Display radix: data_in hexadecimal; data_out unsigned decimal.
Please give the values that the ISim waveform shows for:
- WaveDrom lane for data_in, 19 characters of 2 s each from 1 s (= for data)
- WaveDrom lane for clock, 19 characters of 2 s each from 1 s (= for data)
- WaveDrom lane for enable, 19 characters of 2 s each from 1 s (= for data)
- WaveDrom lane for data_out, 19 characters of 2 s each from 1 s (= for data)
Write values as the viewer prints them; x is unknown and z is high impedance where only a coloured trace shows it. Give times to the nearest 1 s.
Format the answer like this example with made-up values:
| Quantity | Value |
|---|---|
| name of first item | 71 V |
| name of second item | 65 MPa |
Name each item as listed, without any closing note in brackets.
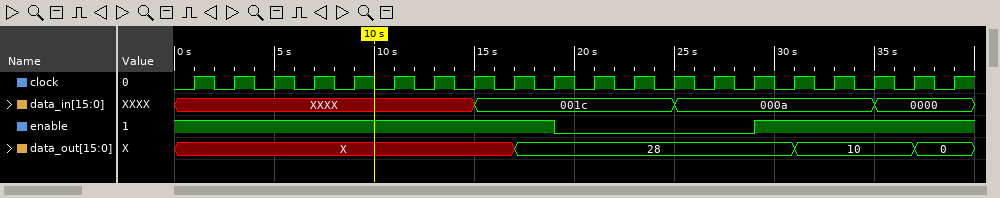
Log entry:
| Quantity | Value |
|---|---|
| WaveDrom lane for data_in, 19 characters of 2 s each from 1 s | {name: 'data_in', wave: 'x......=....=....=.', data: '001c 000a 0000'} |
| WaveDrom lane for clock, 19 characters of 2 s each from 1 s | {name: 'clock', wave: 'p..................'} |
| WaveDrom lane for enable, 19 characters of 2 s each from 1 s | {name: 'enable', wave: '1........0....1....'} |
| WaveDrom lane for data_out, 19 characters of 2 s each from 1 s | {name: 'data_out', wave: 'x.......=......=..=', data: '28 10 0'} |
